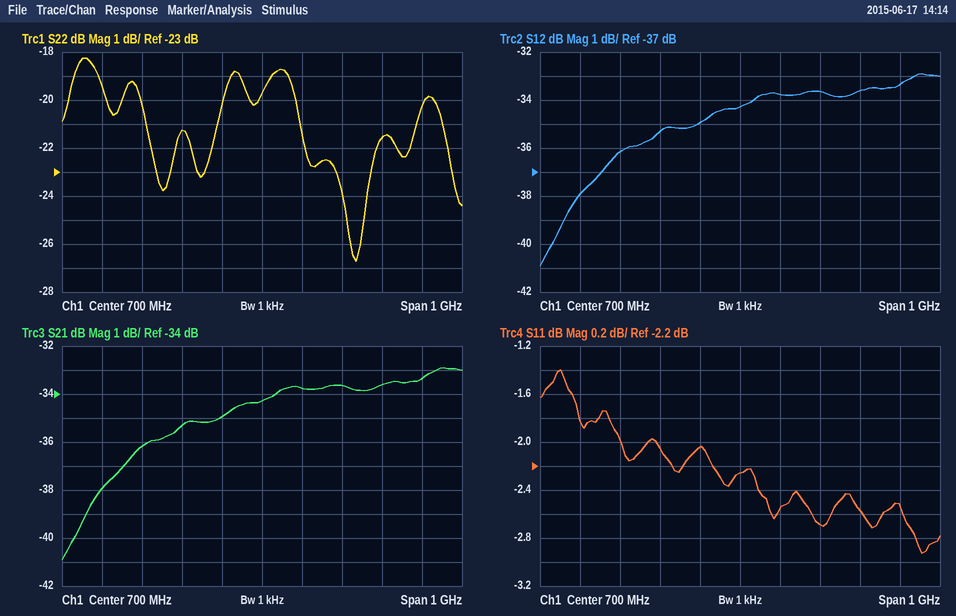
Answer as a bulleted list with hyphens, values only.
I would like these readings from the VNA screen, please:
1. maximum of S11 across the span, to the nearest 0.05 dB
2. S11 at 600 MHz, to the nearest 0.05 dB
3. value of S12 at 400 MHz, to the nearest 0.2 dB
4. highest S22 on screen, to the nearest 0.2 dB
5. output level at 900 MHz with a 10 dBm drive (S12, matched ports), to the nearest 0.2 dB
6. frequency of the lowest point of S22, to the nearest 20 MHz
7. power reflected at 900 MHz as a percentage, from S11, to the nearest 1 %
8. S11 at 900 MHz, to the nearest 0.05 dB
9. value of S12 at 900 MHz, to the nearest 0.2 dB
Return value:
- -1.40 dB
- -2.05 dB
- -36.2 dB
- -18.2 dB
- -23.6 dBm
- 940 MHz
- 54 %
- -2.70 dB
- -33.6 dB
